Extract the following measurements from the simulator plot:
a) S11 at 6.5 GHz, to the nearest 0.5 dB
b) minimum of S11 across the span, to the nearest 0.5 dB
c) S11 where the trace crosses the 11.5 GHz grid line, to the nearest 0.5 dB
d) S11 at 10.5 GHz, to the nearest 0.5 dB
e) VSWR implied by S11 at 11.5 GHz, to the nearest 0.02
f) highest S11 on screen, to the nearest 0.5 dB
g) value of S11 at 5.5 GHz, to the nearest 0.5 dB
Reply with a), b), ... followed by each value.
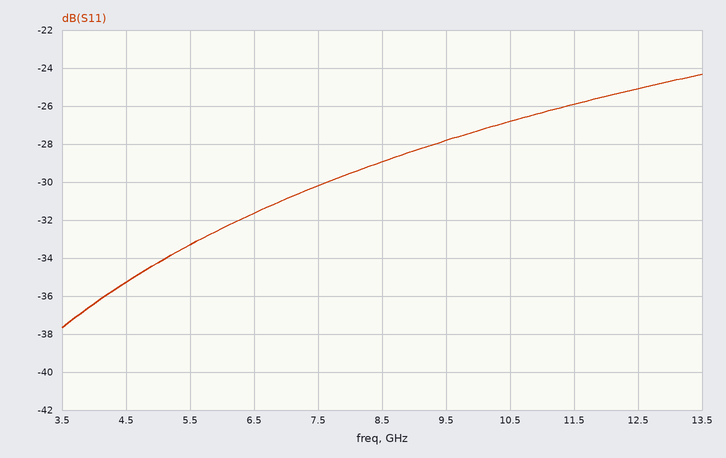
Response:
a) -31.5 dB
b) -37.5 dB
c) -26.0 dB
d) -27.0 dB
e) 1.10
f) -24.5 dB
g) -33.5 dB
